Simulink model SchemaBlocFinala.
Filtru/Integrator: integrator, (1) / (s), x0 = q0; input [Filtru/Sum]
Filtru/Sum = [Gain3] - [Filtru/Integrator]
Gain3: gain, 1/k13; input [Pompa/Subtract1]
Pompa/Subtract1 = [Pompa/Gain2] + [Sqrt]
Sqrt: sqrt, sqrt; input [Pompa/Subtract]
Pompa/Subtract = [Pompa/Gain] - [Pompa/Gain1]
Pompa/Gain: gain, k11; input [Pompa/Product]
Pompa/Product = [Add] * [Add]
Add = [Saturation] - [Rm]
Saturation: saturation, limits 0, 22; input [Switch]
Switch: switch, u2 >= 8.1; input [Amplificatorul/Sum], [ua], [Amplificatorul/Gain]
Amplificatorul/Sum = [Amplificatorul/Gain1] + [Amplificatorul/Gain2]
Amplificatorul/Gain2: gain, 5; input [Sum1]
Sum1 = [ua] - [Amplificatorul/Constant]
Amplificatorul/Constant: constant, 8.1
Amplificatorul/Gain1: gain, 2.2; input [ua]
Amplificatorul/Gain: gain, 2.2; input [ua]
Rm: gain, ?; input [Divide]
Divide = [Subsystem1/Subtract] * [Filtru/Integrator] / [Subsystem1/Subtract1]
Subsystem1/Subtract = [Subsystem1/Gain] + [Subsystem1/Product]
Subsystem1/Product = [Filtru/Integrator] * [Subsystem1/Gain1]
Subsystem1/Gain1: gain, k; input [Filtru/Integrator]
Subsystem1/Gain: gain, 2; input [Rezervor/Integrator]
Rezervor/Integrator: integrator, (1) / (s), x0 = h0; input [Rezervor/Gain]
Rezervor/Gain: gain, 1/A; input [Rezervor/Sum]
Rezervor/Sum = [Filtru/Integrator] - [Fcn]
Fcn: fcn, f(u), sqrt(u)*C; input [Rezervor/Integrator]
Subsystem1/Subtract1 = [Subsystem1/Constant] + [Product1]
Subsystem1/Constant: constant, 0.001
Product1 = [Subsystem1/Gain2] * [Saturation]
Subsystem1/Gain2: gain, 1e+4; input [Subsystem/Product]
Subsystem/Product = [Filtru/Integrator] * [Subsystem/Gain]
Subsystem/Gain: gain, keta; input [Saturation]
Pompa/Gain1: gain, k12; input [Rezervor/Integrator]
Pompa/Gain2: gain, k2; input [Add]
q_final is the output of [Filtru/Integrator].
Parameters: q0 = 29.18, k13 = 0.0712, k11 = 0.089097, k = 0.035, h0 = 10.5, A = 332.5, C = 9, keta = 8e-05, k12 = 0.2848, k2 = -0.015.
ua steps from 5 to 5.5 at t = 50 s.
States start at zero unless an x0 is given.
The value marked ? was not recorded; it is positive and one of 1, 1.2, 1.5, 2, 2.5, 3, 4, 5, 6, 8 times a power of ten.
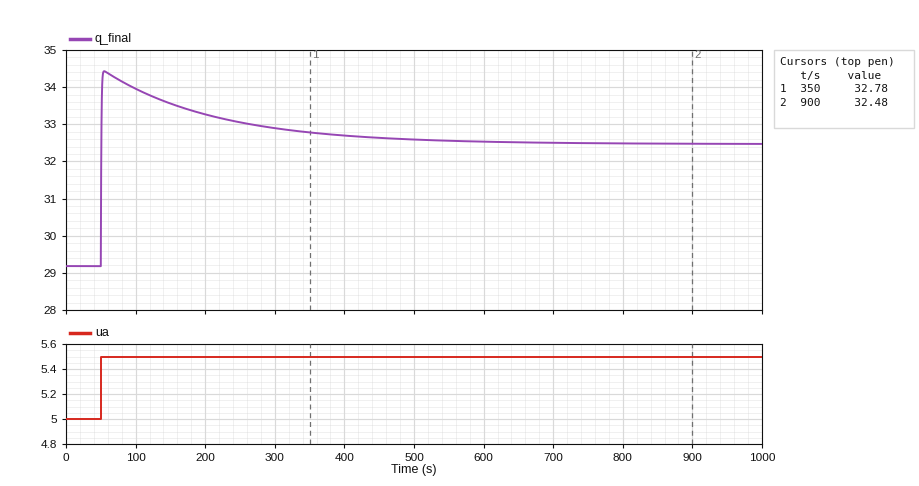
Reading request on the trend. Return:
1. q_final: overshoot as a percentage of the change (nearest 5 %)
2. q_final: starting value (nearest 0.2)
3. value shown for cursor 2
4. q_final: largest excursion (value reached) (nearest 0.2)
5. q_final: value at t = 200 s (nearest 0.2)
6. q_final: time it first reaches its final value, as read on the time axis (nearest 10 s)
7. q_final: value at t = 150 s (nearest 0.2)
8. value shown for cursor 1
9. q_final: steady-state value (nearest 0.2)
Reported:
60 %
29.2
32.48
34.4
33.2
50 s
33.6
32.78
32.4
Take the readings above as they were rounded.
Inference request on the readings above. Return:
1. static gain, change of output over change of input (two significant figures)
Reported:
6.4
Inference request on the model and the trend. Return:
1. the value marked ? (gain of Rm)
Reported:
3
